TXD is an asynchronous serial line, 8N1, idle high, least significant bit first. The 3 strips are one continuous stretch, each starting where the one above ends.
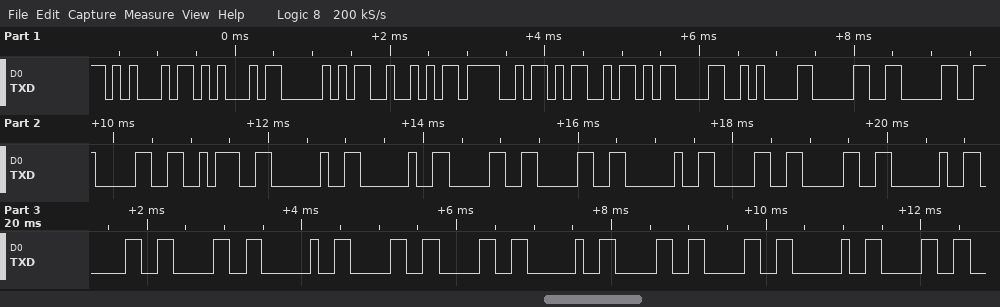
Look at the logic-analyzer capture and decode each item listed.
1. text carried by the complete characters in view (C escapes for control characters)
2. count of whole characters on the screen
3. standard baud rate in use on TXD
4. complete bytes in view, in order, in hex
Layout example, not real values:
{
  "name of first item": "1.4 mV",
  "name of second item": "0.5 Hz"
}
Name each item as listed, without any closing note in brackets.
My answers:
{
  "text carried by the complete characters in view": "\"EEPROM\\r\\n000:  00 00 00 00 00 0\"",
  "count of whole characters on the screen": "30",
  "standard baud rate in use on TXD": "9600 baud",
  "complete bytes in view, in order, in hex": "45 45 50 52 4F 4D 0D 0A 30 30 30 3A 20 20 30 30 20 30 30 20 30 30 20 30 30 20 30 30 20 30"
}
